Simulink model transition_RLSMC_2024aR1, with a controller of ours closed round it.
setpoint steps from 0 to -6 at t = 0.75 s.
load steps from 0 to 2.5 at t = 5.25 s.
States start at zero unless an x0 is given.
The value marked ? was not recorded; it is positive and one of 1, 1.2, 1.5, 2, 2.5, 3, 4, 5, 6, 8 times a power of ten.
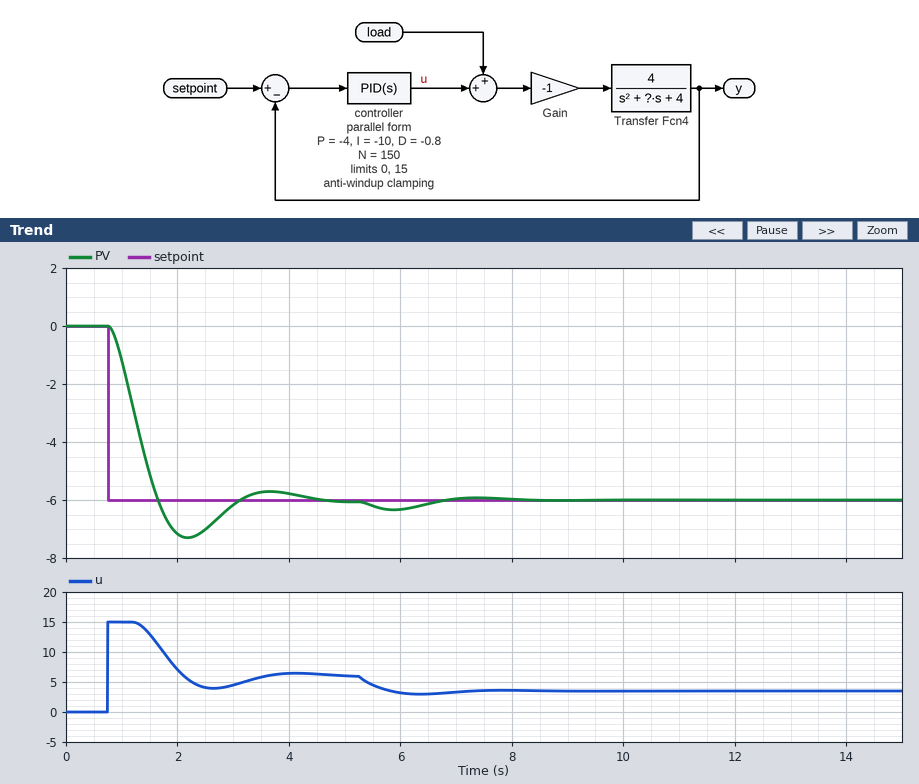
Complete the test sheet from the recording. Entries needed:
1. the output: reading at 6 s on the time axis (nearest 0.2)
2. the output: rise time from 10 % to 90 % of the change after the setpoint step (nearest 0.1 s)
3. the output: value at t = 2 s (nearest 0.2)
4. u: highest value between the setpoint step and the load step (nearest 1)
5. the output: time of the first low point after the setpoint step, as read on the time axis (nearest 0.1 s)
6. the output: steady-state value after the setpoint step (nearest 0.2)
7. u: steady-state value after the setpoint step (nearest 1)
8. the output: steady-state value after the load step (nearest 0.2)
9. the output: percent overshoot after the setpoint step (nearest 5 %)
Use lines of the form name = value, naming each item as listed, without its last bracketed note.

the output: reading at 6 s on the time axis = -6.4
the output: rise time from 10 % to 90 % of the change after the setpoint step = 0.6 s
the output: value at t = 2 s = -7.2
u: highest value between the setpoint step and the load step = 15
the output: time of the first low point after the setpoint step, as read on the time axis = 2.2 s
the output: steady-state value after the setpoint step = -6.0
u: steady-state value after the setpoint step = 6
the output: steady-state value after the load step = -6.0
the output: percent overshoot after the setpoint step = 20 %
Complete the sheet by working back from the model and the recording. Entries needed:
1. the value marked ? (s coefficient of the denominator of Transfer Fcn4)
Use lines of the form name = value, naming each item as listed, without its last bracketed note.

the value marked ? = 6
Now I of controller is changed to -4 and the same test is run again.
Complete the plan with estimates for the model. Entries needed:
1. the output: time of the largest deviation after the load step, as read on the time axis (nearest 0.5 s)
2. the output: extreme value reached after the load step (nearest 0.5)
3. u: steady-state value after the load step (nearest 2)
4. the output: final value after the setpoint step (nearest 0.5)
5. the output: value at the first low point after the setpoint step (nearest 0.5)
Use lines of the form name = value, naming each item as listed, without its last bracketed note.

the output: time of the largest deviation after the load step, as read on the time axis = 6.0 s
the output: extreme value reached after the load step = -6.5
u: steady-state value after the load step = 4
the output: final value after the setpoint step = -6.0
the output: value at the first low point after the setpoint step = -6.5
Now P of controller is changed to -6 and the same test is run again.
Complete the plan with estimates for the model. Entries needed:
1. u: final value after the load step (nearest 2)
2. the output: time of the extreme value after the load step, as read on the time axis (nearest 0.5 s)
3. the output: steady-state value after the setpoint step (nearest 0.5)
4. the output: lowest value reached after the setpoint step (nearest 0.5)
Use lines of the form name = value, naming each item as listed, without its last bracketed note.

u: final value after the load step = 4
the output: time of the extreme value after the load step, as read on the time axis = 6.0 s
the output: steady-state value after the setpoint step = -6.0
the output: lowest value reached after the setpoint step = -6.5
